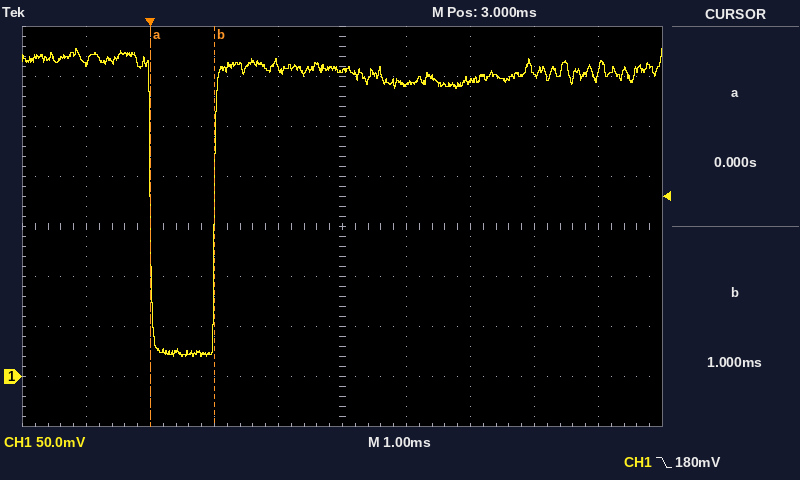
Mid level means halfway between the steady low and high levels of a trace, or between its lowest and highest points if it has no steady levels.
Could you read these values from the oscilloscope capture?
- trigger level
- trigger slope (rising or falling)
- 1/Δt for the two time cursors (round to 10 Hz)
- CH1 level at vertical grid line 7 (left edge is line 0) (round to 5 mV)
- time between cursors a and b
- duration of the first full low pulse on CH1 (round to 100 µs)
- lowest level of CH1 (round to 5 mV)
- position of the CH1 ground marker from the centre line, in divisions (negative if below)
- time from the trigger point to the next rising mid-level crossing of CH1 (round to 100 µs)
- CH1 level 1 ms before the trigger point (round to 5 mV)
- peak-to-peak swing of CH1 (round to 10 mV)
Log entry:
180 mV
falling
1.00 kHz
295 mV
1.0 ms
1.0 ms
20 mV
-3.0 div
1.0 ms
315 mV
310 mV
